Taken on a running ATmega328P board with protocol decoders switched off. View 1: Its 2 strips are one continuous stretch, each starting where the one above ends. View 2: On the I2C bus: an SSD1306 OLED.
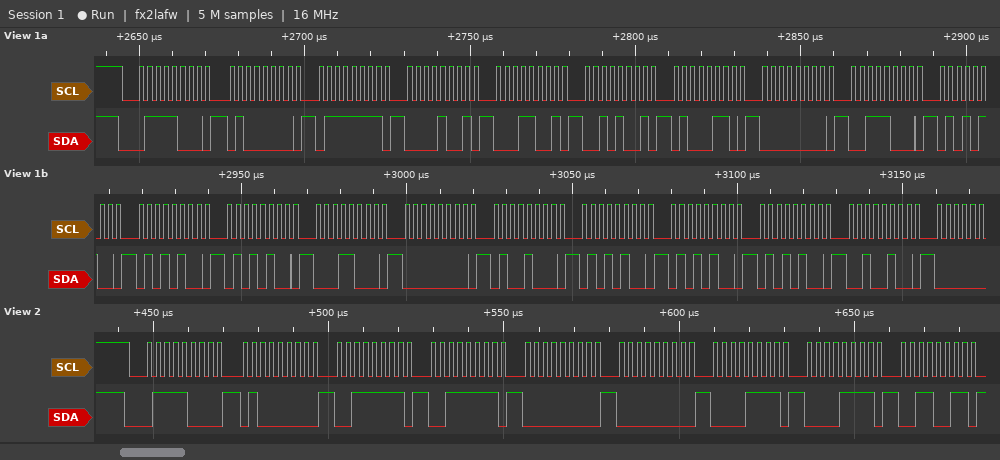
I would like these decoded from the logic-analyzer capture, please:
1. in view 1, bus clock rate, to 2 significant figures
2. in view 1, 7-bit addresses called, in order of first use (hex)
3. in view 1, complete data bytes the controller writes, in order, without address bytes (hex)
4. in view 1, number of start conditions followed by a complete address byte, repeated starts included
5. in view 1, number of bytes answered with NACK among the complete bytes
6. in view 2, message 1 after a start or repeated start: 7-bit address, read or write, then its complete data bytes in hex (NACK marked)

400 kHz
0x3C
40 7F 09 19 29 46 00 38 54 54 54 18 00 48 54 54 54 24
1
0
0x3C write: 40 3F 3F 00 00 0F 0F 33
